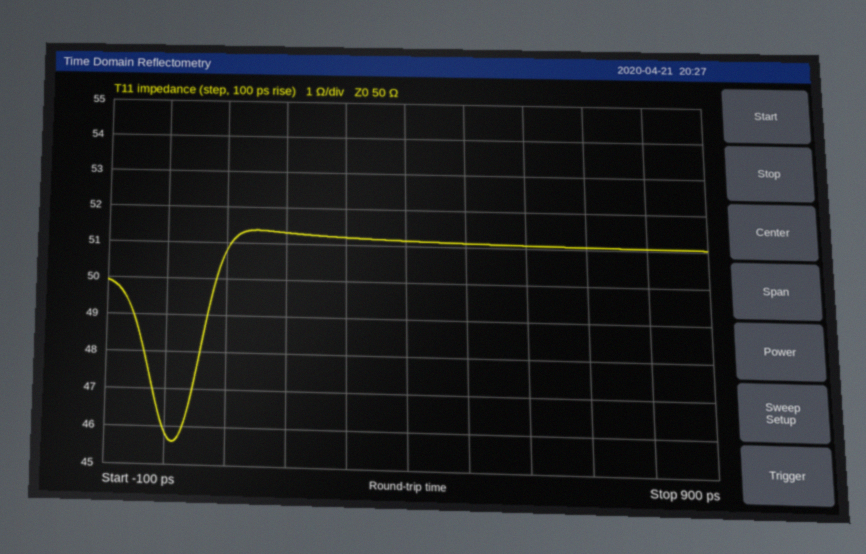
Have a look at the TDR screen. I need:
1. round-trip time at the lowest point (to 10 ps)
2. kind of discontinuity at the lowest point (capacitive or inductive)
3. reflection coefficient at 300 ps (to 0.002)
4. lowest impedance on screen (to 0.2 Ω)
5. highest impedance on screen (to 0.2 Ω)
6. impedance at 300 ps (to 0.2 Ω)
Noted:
10 ps
capacitive
+0.012
45.6 Ω
51.4 Ω
51.2 Ω
